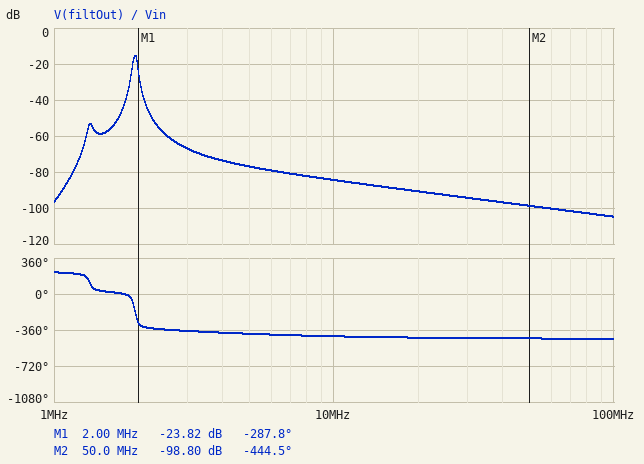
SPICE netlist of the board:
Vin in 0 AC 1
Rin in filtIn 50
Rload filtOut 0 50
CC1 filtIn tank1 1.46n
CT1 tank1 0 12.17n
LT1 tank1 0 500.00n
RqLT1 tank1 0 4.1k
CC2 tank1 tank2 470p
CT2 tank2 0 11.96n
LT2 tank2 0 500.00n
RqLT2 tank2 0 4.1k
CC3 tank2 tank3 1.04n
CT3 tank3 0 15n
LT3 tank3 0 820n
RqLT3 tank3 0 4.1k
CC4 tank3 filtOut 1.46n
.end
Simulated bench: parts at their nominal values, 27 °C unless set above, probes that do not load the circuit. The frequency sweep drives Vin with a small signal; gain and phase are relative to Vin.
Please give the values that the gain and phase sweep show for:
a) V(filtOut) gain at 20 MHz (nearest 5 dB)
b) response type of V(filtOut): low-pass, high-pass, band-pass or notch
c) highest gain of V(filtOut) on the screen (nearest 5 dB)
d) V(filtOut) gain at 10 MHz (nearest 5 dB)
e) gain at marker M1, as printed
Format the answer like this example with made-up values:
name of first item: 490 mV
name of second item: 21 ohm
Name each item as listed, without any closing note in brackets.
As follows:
V(filtOut) gain at 20 MHz: -90 dB
response type of V(filtOut): low-pass, high-pass, band-pass or notch: band-pass
highest gain of V(filtOut) on the screen: -15 dB
V(filtOut) gain at 10 MHz: -85 dB
gain at marker M1, as printed: -23.82 dB
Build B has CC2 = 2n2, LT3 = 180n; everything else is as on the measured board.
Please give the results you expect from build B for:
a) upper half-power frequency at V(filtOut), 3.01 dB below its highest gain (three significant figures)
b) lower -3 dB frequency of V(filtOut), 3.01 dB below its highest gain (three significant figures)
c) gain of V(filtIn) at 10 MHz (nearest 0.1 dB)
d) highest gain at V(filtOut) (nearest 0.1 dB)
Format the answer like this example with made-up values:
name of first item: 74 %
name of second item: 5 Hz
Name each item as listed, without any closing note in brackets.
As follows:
upper half-power frequency at V(filtOut), 3.01 dB below its highest gain: 2.00 MHz
lower -3 dB frequency of V(filtOut), 3.01 dB below its highest gain: 1.94 MHz
gain of V(filtIn) at 10 MHz: -12.6 dB
highest gain at V(filtOut): -26.0 dB
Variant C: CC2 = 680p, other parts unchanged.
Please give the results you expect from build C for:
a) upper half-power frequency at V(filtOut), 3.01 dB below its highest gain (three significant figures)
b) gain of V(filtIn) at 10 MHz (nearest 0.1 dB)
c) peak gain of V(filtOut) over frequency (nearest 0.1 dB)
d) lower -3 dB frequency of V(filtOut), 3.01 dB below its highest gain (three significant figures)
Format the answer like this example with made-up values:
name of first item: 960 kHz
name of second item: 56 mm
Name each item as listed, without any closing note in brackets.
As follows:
upper half-power frequency at V(filtOut), 3.01 dB below its highest gain: 1.99 MHz
gain of V(filtIn) at 10 MHz: -12.5 dB
peak gain of V(filtOut) over frequency: -17.3 dB
lower -3 dB frequency of V(filtOut), 3.01 dB below its highest gain: 1.88 MHz
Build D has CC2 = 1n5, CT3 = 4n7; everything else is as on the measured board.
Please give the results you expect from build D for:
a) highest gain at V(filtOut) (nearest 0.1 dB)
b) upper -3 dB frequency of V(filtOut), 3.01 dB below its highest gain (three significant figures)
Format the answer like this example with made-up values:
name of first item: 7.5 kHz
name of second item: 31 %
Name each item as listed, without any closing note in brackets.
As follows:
highest gain at V(filtOut): -8.3 dB
upper -3 dB frequency of V(filtOut), 3.01 dB below its highest gain: 1.99 MHz
